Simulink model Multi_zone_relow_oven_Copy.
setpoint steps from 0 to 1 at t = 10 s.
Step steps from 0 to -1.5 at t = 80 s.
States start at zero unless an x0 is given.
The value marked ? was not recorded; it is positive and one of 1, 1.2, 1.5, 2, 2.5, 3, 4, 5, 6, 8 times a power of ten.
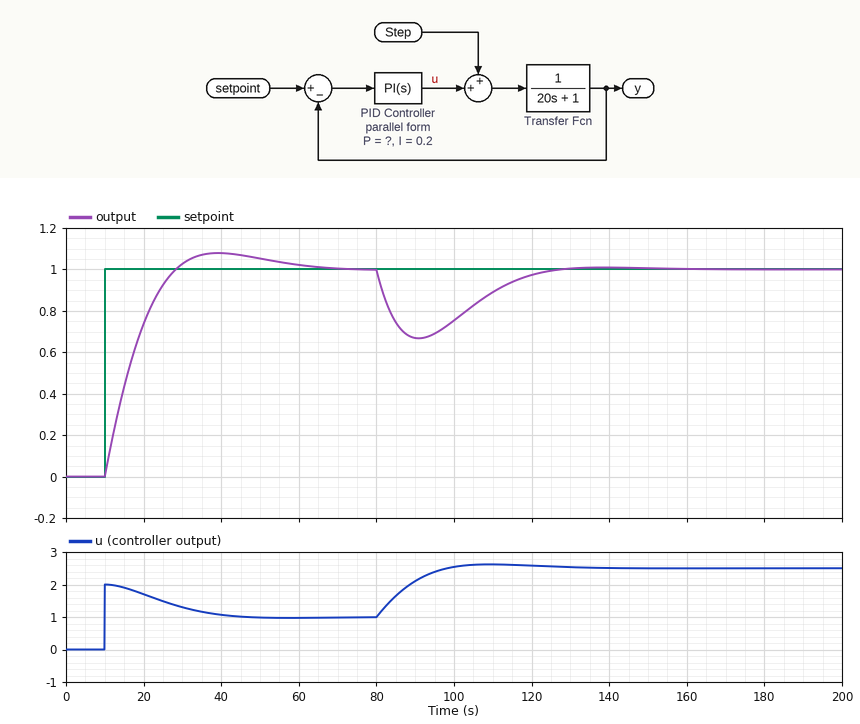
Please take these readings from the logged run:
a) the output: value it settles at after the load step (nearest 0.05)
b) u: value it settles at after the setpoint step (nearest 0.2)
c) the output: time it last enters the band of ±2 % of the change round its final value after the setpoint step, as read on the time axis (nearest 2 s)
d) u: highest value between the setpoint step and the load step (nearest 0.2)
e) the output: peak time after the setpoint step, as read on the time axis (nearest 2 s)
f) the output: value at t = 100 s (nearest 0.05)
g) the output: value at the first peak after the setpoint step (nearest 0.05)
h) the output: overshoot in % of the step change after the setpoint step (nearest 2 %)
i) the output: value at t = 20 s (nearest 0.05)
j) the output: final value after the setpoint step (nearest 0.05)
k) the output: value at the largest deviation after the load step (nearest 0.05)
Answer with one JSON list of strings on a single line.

["1.00", "1.0", "60 s", "2.0", "40 s", "0.75", "1.10", "8 %", "0.75", "1.00", "0.65"]
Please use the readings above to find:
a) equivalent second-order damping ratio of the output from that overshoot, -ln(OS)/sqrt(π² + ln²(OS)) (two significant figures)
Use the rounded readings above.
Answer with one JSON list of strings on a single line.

["0.63"]
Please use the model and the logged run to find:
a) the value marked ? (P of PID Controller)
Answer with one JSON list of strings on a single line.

["2"]
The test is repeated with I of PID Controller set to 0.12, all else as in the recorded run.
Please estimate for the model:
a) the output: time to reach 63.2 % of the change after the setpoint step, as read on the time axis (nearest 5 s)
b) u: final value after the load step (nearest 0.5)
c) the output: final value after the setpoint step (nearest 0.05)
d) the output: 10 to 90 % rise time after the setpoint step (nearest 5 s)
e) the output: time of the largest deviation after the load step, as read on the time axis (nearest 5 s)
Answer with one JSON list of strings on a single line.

["20 s", "2.5", "1.00", "20 s", "95 s"]
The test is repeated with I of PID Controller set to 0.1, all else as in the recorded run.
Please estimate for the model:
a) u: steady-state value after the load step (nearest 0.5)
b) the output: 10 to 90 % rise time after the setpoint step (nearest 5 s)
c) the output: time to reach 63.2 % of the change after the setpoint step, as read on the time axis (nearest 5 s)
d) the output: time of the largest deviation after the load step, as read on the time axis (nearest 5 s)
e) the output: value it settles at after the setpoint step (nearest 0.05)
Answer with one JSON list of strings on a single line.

["2.5", "20 s", "20 s", "95 s", "1.00"]
